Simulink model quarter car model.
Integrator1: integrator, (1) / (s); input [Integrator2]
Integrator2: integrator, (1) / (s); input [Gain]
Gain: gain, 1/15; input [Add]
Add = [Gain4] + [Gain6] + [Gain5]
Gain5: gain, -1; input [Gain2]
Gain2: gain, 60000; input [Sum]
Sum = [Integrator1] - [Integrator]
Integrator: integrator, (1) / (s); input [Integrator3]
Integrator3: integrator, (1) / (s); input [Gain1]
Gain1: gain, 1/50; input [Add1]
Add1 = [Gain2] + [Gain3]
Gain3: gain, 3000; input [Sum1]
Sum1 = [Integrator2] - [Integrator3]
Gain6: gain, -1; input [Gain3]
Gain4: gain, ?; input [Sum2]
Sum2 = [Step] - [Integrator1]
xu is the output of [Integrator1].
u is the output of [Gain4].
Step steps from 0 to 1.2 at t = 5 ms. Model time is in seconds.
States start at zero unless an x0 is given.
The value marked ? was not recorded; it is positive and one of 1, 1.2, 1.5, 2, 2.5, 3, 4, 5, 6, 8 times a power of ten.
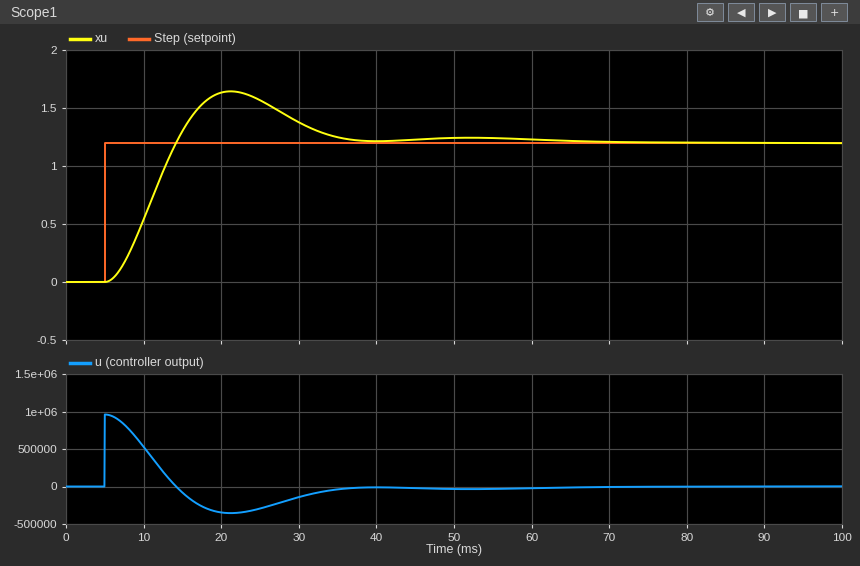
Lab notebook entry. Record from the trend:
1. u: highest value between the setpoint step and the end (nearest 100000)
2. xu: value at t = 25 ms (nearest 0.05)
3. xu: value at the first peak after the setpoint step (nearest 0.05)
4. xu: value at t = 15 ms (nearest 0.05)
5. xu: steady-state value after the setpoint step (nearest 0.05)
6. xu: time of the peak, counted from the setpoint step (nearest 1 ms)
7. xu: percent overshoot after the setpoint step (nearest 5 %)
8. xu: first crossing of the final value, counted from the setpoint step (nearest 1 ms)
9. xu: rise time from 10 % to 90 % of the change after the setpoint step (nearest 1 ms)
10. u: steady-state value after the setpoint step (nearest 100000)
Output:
1000000
1.55
1.65
1.30
1.20
16 ms
35 %
9 ms
6 ms
0
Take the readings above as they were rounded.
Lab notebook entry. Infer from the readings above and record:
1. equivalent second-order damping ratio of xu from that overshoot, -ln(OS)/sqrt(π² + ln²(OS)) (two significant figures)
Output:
0.32
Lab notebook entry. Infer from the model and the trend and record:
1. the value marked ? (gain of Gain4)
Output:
800000
